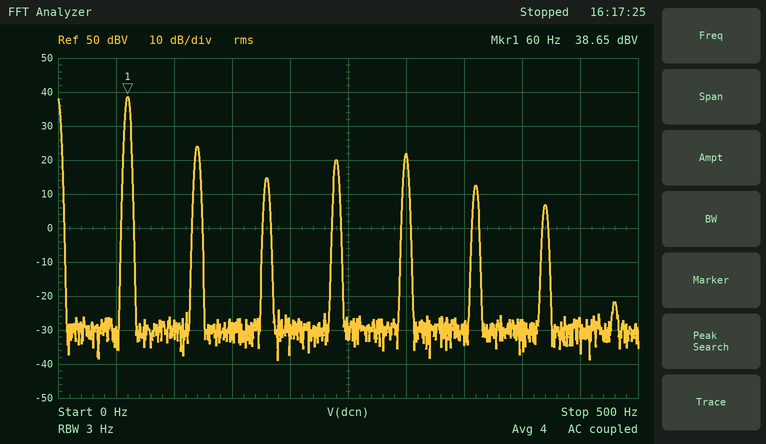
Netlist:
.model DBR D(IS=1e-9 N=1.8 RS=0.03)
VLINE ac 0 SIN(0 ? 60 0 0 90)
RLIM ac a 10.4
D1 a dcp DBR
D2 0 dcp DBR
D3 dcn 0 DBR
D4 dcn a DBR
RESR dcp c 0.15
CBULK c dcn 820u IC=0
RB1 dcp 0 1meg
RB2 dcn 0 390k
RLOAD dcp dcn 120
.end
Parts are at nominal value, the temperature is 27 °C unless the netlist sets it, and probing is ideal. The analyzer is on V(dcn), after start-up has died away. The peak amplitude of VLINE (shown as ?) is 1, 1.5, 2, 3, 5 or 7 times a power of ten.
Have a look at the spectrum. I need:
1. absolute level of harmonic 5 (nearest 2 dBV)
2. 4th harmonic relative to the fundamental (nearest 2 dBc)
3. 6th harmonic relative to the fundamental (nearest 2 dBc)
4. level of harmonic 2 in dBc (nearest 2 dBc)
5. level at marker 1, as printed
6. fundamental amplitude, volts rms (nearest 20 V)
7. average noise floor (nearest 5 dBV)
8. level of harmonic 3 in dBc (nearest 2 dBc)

22 dBV
-18 dBc
-26 dBc
-14 dBc
38.65 dBV
80 V
-30 dBV
-24 dBc
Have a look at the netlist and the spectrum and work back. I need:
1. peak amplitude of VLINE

300 V
